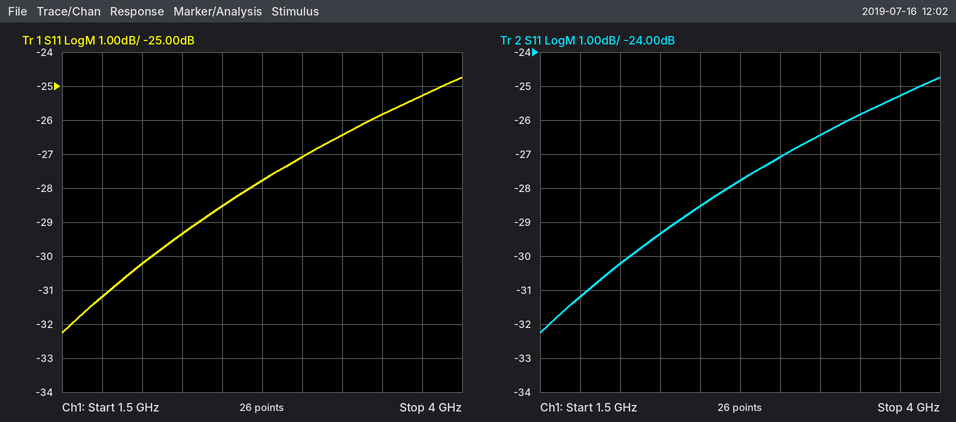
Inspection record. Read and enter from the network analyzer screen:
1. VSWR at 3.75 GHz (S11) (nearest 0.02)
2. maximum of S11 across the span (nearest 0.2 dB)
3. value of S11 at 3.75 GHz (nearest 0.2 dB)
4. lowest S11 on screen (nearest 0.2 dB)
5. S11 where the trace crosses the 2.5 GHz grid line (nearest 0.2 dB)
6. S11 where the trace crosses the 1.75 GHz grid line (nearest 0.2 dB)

1.12
-24.8 dB
-25.2 dB
-32.2 dB
-28.6 dB
-31.2 dB
